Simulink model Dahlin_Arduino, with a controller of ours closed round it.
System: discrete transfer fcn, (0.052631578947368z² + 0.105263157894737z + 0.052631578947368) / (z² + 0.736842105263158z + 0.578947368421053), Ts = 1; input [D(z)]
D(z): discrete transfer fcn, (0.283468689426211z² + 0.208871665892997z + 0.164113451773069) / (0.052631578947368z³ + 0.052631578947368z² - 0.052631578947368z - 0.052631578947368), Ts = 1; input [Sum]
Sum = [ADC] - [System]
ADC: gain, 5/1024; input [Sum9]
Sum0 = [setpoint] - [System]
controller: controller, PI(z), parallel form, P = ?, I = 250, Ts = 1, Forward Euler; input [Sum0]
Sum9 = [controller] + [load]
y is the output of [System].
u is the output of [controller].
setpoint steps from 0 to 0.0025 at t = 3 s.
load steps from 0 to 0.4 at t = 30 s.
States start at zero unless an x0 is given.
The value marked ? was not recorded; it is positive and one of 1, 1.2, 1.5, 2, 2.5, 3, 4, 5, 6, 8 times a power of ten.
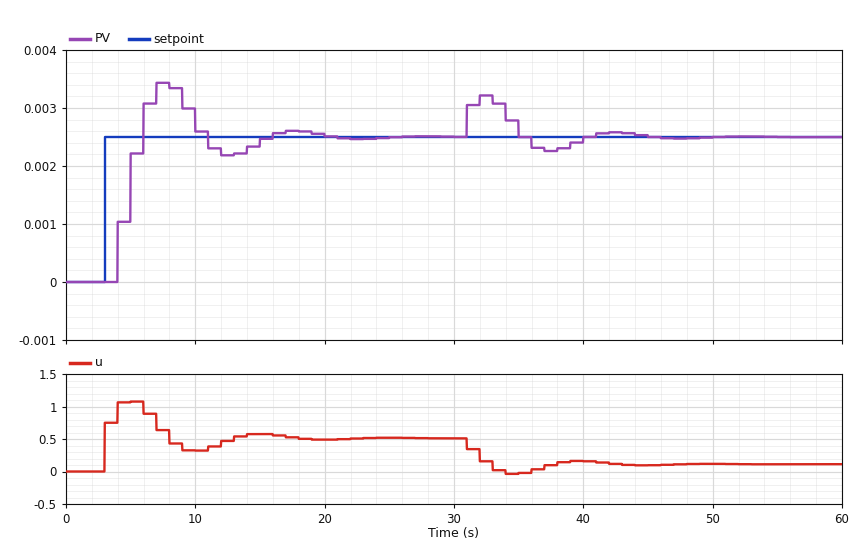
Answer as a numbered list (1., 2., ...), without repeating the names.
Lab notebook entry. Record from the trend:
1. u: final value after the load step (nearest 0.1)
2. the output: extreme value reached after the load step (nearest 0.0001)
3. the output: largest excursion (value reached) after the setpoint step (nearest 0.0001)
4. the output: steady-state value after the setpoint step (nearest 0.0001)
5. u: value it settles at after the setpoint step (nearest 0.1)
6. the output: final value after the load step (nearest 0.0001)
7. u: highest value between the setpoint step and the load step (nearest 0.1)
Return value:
1. 0.1
2. 0.0032
3. 0.0034
4. 0.0025
5. 0.5
6. 0.0025
7. 1.1
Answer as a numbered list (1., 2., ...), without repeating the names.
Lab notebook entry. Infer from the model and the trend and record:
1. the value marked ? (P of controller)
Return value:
1. 300
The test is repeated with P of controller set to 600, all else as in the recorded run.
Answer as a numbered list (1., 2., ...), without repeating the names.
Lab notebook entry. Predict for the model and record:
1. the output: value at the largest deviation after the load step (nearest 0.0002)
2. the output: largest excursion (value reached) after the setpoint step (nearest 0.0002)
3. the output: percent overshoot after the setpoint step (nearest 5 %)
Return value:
1. 0.0030
2. 0.0028
3. 10 %
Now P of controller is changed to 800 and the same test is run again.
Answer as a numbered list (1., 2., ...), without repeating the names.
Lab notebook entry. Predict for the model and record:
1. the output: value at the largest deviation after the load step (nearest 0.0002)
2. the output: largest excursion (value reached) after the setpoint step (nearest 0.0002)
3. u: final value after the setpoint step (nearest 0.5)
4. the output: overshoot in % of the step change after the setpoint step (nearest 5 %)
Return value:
1. 0.0030
2. 0.0028
3. 0.5
4. 10 %
